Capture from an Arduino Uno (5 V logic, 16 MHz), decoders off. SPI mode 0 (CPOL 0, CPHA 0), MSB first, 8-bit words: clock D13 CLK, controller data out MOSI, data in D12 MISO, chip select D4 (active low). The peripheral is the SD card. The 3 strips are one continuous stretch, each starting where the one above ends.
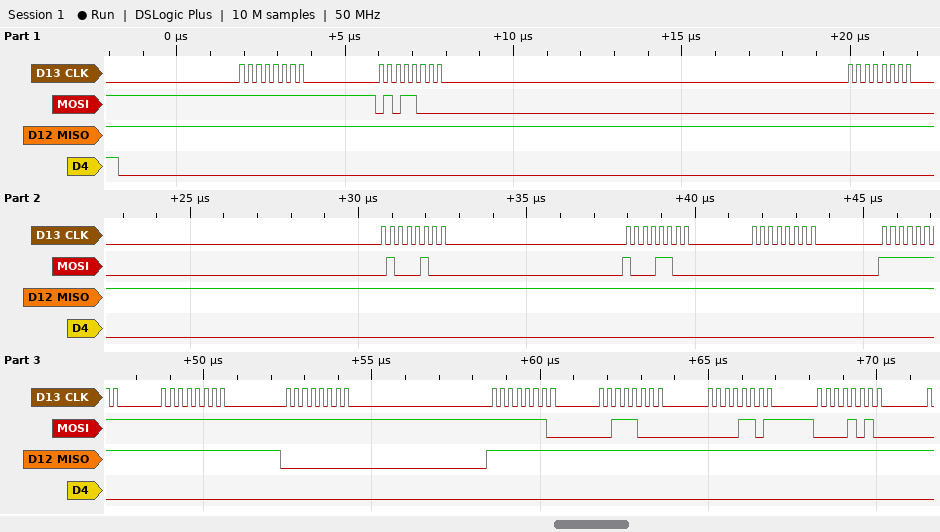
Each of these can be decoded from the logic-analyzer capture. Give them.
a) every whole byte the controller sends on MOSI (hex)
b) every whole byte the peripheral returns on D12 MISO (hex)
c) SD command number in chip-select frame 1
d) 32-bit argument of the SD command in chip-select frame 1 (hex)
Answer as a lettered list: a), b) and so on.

a) FF 58 00 44 8C 00 FF FF FF FE 38 0D 0A
b) FF FF FF FF FF FF FF FF 00 FF FF FF FF
c) CMD24
d) 0x00448C00
